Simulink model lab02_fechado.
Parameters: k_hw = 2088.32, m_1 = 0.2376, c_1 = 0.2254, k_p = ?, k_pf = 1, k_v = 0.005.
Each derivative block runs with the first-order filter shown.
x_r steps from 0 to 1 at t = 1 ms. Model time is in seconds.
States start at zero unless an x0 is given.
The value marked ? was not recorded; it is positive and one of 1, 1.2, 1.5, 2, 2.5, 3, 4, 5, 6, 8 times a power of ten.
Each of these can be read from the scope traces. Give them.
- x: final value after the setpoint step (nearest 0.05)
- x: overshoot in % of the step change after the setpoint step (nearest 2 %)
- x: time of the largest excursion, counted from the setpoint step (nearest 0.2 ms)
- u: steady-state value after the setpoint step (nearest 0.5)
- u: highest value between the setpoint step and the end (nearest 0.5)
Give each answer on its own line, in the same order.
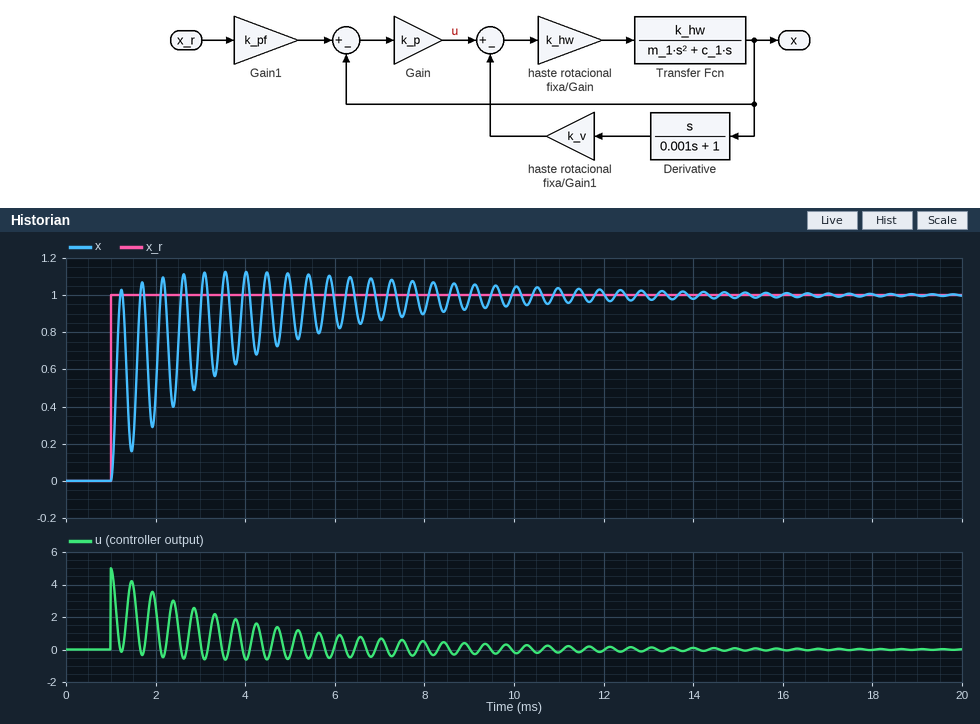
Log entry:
1.00
12 %
2.6 ms
0.0
5.0
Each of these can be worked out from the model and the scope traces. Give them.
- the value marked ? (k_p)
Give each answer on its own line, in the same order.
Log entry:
5
